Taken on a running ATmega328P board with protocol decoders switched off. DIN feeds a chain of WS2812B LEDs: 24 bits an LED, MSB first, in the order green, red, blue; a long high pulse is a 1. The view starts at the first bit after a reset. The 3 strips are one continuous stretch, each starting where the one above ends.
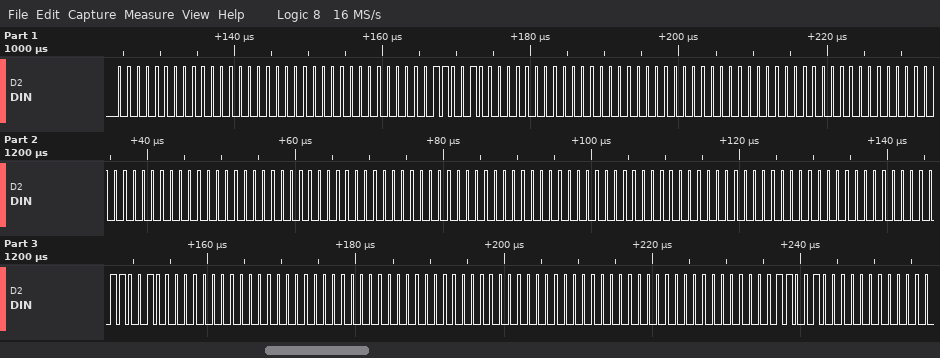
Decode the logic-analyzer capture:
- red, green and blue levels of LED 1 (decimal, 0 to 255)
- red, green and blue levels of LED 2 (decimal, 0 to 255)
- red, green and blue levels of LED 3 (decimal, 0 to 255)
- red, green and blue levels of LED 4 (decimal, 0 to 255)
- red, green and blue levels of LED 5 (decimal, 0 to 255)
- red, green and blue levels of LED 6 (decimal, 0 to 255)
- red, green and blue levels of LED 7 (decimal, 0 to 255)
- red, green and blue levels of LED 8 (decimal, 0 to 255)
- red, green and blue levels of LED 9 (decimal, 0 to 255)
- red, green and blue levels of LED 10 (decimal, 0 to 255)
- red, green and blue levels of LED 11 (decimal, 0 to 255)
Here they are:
0, 0, 0
50, 0, 0
0, 0, 0
0, 0, 0
0, 0, 0
0, 0, 0
0, 0, 0
50, 0, 0
0, 0, 0
0, 0, 0
50, 0, 0
